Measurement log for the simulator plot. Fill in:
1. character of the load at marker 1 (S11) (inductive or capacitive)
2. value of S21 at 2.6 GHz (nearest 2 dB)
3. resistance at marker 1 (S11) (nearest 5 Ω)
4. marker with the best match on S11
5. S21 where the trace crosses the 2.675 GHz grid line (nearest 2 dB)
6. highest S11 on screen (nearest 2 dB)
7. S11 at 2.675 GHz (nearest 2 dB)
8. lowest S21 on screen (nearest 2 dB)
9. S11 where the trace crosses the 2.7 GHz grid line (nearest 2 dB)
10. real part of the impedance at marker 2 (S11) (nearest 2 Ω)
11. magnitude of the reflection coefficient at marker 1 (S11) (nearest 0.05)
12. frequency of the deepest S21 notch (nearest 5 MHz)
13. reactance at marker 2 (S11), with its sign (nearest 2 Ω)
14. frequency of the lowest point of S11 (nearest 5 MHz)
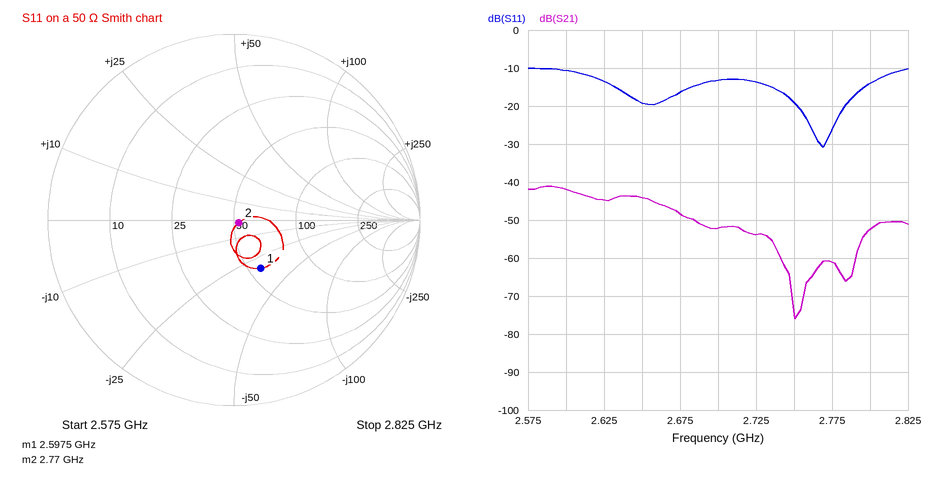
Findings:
capacitive
-42 dB
55 Ω
marker 2
-48 dB
-10 dB
-16 dB
-76 dB
-14 dB
52 Ω
0.30
2.750 GHz
-2 Ω
2.770 GHz
